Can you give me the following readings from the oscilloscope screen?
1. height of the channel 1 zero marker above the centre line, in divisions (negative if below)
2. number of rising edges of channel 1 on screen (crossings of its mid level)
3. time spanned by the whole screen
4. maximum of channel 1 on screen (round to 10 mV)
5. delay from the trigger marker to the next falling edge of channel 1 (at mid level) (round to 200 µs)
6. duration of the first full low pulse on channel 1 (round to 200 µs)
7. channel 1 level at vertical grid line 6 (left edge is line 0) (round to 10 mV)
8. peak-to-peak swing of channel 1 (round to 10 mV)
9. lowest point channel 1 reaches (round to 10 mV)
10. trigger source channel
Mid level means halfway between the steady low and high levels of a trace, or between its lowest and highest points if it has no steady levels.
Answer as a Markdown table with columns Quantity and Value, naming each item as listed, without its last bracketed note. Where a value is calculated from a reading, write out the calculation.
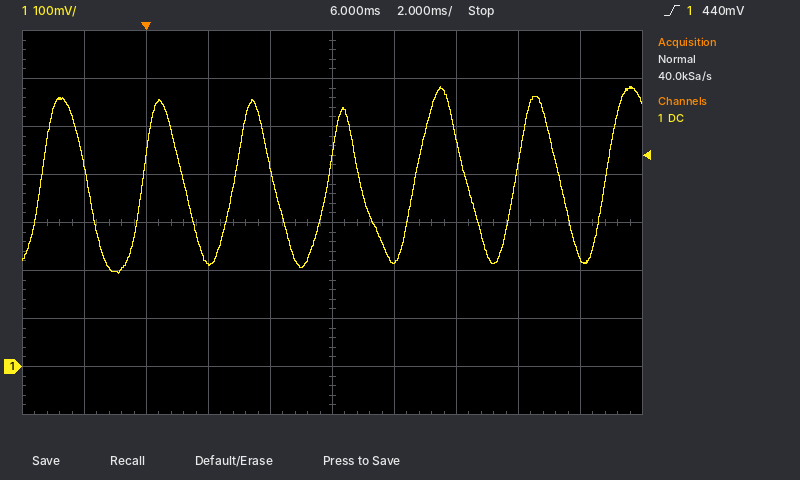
| Quantity | Value |
|---|---|
| height of the channel 1 zero marker above the centre line, in divisions | -3.0 div |
| number of rising edges of channel 1 on screen | 7 |
| time spanned by the whole screen | 20 ms |
| maximum of channel 1 on screen | 580 mV |
| delay from the trigger marker to the next falling edge of channel 1 (at mid level) | 1.2 ms |
| duration of the first full low pulse on channel 1 | 1.8 ms |
| channel 1 level at vertical grid line 6 (left edge is line 0) | 220 mV |
| peak-to-peak swing of channel 1 | 580 mV − (190 mV) = 390 mV |
| lowest point channel 1 reaches | 190 mV |
| trigger source channel | channel 1 |
